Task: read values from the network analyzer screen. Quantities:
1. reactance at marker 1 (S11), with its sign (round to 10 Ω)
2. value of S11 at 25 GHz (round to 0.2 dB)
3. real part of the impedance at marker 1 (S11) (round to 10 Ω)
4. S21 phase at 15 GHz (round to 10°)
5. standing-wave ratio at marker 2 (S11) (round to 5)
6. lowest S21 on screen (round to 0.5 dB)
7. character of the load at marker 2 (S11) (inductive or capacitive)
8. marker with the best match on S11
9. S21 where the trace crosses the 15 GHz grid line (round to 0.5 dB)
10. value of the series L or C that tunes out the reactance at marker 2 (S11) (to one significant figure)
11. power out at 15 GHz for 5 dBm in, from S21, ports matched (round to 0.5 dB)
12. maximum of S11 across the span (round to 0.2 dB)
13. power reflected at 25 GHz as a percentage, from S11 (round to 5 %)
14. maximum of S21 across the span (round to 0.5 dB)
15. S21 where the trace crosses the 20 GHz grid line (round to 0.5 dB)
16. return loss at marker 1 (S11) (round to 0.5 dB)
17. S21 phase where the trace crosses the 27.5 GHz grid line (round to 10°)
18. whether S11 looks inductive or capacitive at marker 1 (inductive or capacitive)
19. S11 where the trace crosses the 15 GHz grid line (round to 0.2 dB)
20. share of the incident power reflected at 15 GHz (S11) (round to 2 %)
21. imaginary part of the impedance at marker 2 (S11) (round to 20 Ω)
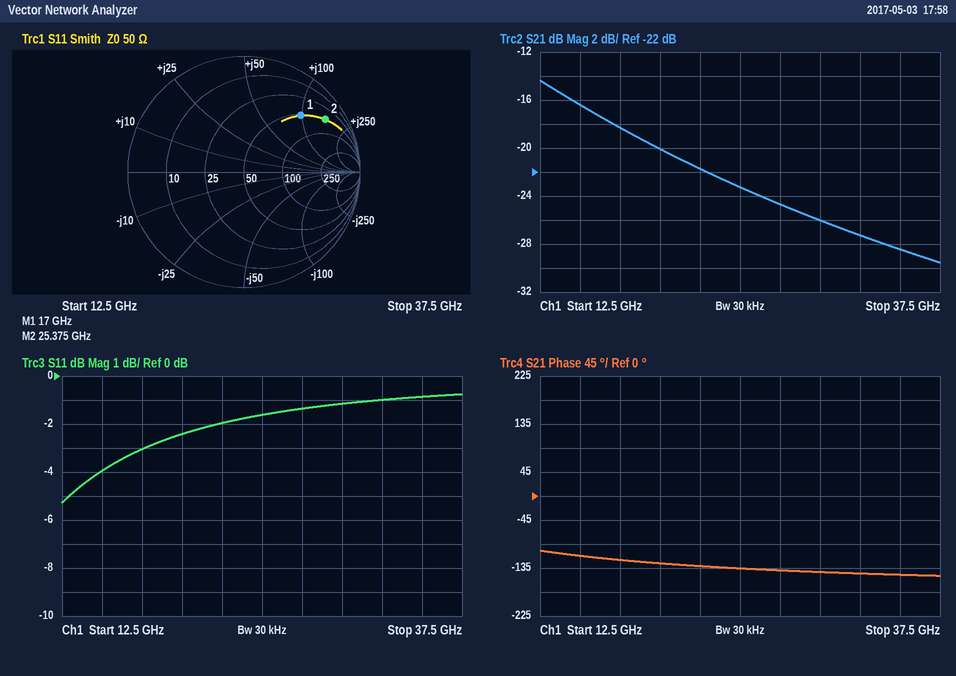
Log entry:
+100 Ω
-1.6 dB
50 Ω
-110°
10
-29.5 dB
inductive
marker 1
-16.5 dB
40 fF
-11.5 dBm
-0.8 dB
70 %
-14.5 dB
-20.0 dB
3.0 dB
-140°
inductive
-4.0 dB
40 %
+160 Ω
